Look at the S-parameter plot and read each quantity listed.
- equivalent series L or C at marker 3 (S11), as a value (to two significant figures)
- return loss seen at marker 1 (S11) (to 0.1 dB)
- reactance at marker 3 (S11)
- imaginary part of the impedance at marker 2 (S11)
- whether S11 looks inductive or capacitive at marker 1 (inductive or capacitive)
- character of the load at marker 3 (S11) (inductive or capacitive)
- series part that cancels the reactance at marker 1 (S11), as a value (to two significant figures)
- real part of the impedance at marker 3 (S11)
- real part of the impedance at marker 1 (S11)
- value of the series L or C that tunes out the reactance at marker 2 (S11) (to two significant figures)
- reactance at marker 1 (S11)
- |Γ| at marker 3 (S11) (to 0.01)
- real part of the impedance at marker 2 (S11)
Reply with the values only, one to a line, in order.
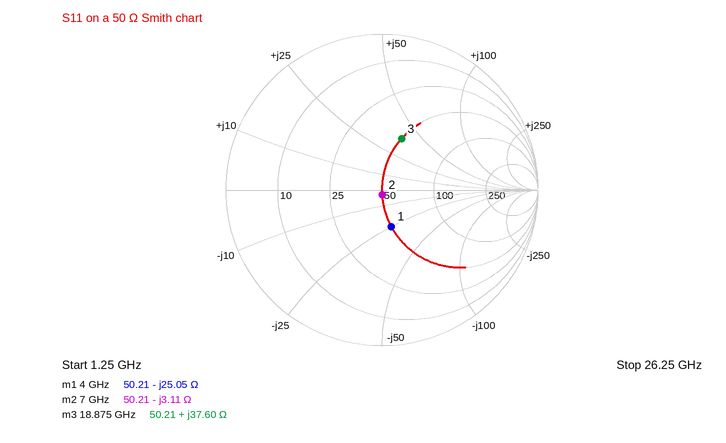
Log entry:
320 pH
12.3 dB
+37.60 Ω
-3.11 Ω
capacitive
inductive
1.00 nH
50.21 Ω
50.21 Ω
71 pH
-25.05 Ω
0.35
50.21 Ω
